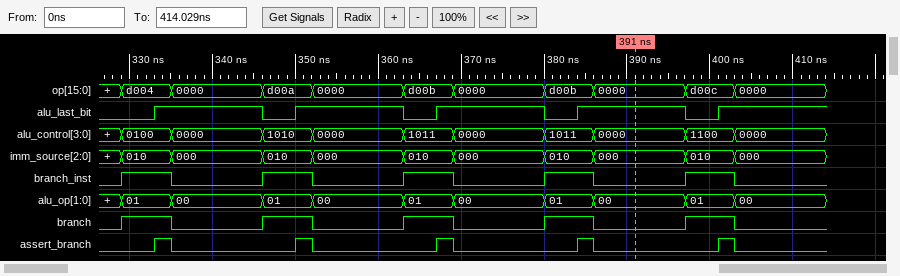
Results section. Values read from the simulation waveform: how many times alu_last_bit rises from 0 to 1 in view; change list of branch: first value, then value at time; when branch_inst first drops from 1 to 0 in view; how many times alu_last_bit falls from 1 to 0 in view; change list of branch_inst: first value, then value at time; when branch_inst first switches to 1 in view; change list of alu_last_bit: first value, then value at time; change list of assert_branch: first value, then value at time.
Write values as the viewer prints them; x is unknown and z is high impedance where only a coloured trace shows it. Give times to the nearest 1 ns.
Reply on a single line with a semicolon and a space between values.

5; 0, 1 at 329 ns, 0 at 335 ns, 1 at 346 ns, 0 at 352 ns, 1 at 363 ns, 0 at 369 ns, 1 at 380 ns, 0 at 386 ns, 1 at 397 ns, 0 at 403 ns; 335 ns; 4; 0, 1 at 329 ns, 0 at 335 ns, 1 at 346 ns, 0 at 352 ns, 1 at 363 ns, 0 at 369 ns, 1 at 380 ns, 0 at 386 ns, 1 at 397 ns, 0 at 403 ns; 329 ns; 0, 1 at 333 ns, 0 at 346 ns, 1 at 350 ns, 0 at 363 ns, 1 at 367 ns, 0 at 380 ns, 1 at 384 ns, 0 at 397 ns, 1 at 401 ns; 0, 1 at 333 ns, 0 at 335 ns, 1 at 350 ns, 0 at 352 ns, 1 at 367 ns, 0 at 369 ns, 1 at 384 ns, 0 at 386 ns, 1 at 401 ns, 0 at 403 ns
